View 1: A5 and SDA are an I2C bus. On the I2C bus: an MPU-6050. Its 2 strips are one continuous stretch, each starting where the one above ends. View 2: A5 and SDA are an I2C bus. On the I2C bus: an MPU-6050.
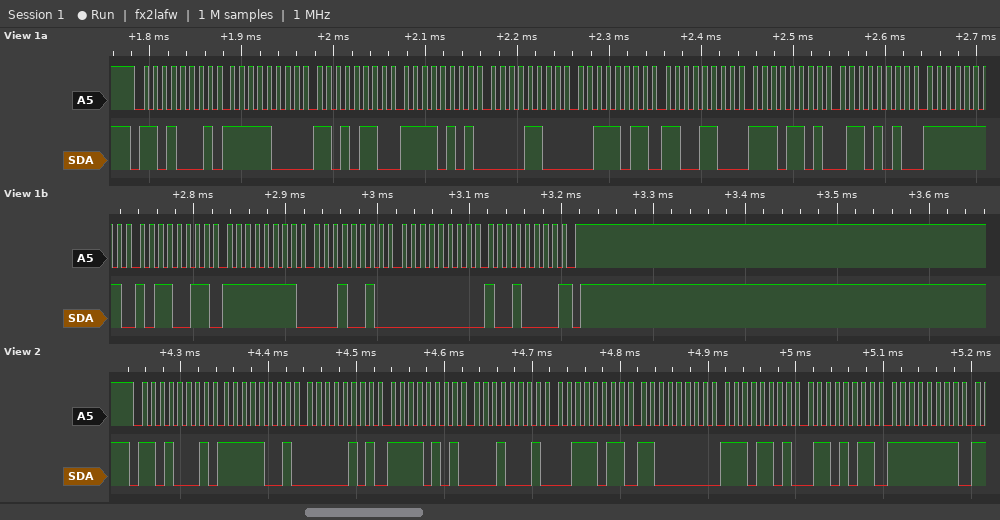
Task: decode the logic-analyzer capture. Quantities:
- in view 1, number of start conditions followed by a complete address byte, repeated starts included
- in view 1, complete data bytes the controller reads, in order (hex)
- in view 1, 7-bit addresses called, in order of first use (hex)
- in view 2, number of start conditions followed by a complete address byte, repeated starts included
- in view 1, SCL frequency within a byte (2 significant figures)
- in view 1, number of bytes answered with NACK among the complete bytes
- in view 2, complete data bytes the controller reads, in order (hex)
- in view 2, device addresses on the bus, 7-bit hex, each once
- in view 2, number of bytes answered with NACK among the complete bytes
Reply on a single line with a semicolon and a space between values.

1; F8 D6 F5 0C 3B CC ED 6A FF B3 FF 12 00 90; 0x68; 1; 100 kHz; 1; F9 05 F5 11 3B C0 ED 6B FF; 0x68; 0
